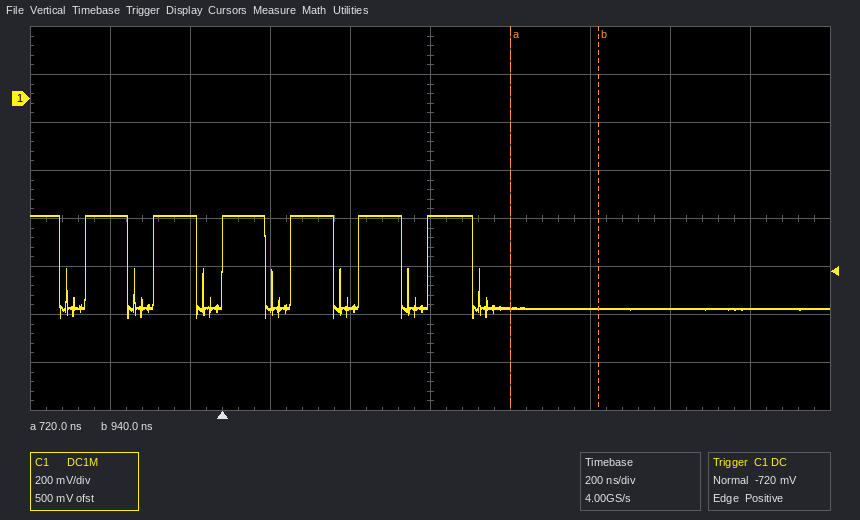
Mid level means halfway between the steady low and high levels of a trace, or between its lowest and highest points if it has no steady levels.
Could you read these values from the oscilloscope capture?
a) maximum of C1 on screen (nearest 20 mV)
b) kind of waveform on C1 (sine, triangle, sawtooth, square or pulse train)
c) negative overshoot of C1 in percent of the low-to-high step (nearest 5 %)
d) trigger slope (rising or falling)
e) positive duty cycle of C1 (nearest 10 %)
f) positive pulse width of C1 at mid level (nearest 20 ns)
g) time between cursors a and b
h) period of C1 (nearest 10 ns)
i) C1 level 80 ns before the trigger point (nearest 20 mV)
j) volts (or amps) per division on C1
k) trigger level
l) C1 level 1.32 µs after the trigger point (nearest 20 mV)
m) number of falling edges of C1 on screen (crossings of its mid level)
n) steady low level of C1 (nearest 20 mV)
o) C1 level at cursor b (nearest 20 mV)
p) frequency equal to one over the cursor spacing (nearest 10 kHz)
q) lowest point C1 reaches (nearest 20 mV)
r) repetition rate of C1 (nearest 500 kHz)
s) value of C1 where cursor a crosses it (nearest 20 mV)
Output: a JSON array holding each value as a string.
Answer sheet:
["-480 mV", "pulse train", "10 %", "rising", "60 %", "100 ns", "220 ns", "170 ns", "-480 mV", "200 mV", "-720 mV", "-880 mV", "7", "-880 mV", "-880 mV", "4.55 MHz", "-920 mV", "6.0 MHz", "-880 mV"]
